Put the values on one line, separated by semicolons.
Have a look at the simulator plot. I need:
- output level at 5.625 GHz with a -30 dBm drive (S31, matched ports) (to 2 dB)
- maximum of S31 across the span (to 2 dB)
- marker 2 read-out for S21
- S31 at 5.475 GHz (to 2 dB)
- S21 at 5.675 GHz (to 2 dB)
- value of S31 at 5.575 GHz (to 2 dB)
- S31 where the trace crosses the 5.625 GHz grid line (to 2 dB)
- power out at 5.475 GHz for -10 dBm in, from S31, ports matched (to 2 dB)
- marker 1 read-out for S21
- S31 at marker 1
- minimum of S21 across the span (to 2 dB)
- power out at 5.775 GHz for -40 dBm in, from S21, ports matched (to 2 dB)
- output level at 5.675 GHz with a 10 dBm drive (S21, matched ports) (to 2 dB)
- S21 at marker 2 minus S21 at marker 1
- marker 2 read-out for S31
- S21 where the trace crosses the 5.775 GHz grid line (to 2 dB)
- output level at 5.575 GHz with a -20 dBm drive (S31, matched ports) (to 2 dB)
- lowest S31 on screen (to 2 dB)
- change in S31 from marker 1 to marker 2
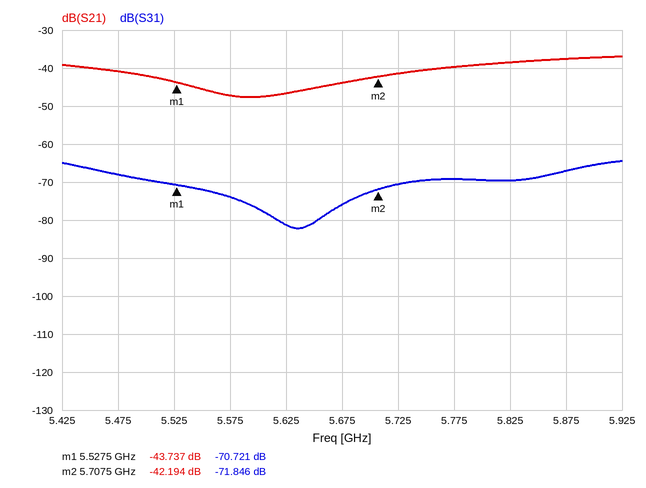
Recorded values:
-112 dBm; -64 dB; -42.194 dB; -68 dB; -44 dB; -74 dB; -82 dB; -78 dBm; -43.737 dB; -70.721 dB; -48 dB; -80 dBm; -34 dBm; 1.543 dB; -71.846 dB; -40 dB; -94 dBm; -82 dB; -1.125 dB
